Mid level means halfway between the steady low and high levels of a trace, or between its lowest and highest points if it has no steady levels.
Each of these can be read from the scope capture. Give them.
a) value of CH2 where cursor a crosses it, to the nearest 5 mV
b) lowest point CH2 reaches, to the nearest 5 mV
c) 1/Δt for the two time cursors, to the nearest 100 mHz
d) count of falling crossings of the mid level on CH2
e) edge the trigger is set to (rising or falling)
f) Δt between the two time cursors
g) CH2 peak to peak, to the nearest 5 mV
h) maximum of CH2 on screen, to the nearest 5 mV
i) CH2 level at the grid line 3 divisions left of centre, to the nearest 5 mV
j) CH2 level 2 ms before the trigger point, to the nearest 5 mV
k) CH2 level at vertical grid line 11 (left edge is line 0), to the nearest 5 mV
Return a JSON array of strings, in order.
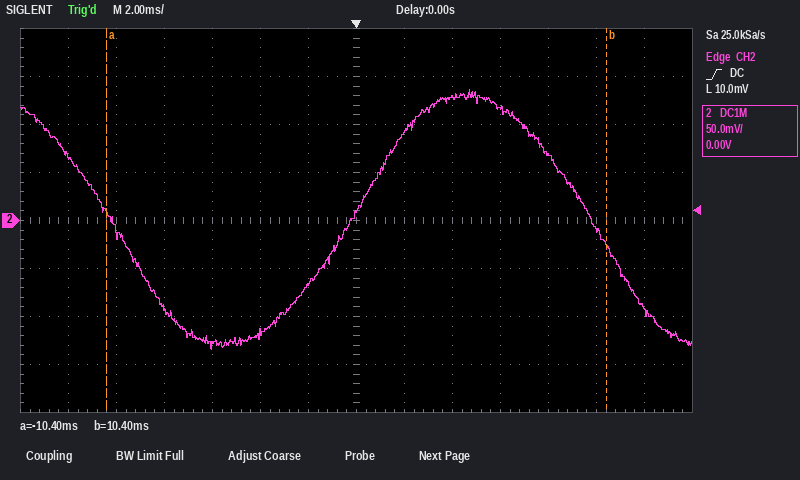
["10 mV", "-135 mV", "48.1 Hz", "2", "rising", "20.8 ms", "270 mV", "135 mV", "-130 mV", "-65 mV", "70 mV"]
